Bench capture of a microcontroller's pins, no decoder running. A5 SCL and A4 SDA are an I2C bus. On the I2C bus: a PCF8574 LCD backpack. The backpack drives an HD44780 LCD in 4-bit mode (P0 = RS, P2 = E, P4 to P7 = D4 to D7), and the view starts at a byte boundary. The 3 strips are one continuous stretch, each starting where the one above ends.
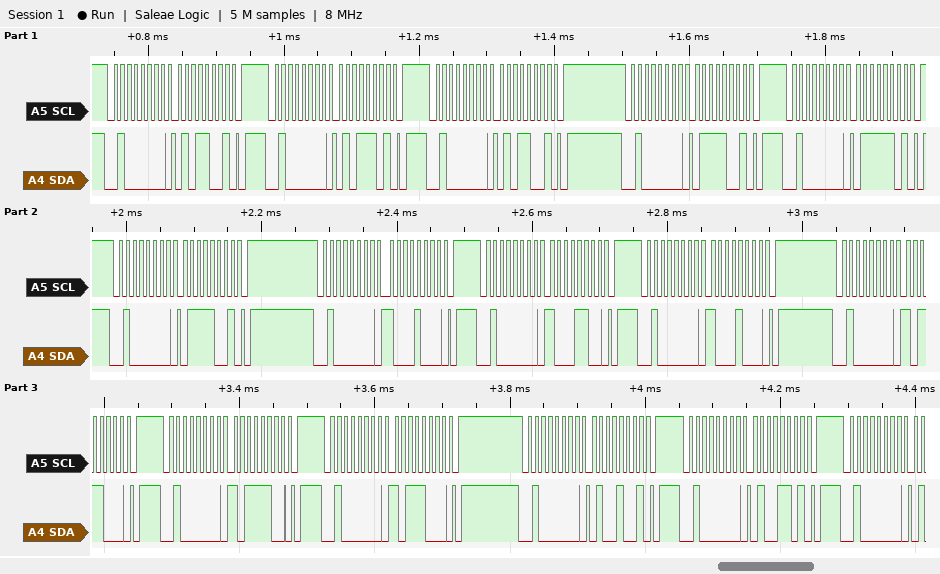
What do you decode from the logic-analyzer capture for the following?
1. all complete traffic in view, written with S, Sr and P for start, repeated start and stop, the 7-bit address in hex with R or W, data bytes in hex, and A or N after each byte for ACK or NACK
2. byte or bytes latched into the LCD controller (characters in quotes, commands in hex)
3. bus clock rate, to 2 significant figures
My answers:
S 20W A 59 A P S 20W A 5D A P S 20W A 59 A P S 20W A 79 A P S 20W A 7D A P S 20W A 79 A P S 20W A 88 A P S 20W A 8C A P S 20W A 88 A P S 20W A B8 A P S 20W A BC A P S 20W A B8 A P S 20W A 49 A P S 20W A 4D A P S 20W A
'W' 0x8B
100 kHz
